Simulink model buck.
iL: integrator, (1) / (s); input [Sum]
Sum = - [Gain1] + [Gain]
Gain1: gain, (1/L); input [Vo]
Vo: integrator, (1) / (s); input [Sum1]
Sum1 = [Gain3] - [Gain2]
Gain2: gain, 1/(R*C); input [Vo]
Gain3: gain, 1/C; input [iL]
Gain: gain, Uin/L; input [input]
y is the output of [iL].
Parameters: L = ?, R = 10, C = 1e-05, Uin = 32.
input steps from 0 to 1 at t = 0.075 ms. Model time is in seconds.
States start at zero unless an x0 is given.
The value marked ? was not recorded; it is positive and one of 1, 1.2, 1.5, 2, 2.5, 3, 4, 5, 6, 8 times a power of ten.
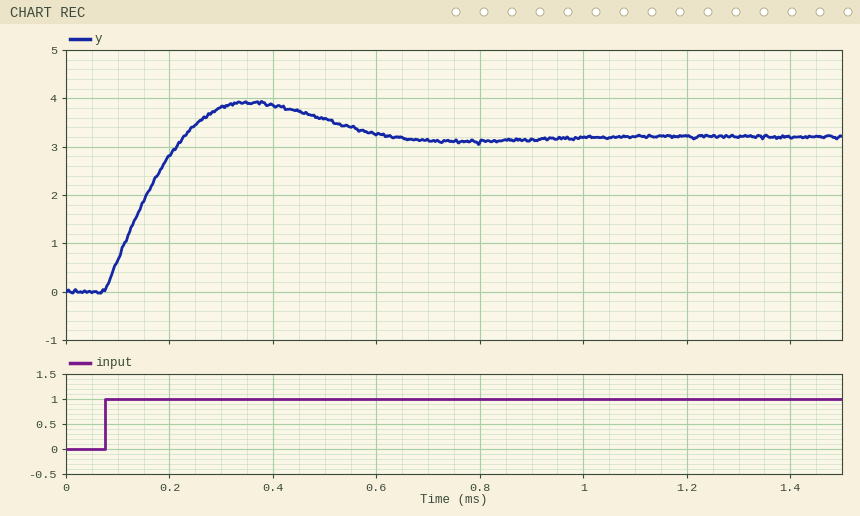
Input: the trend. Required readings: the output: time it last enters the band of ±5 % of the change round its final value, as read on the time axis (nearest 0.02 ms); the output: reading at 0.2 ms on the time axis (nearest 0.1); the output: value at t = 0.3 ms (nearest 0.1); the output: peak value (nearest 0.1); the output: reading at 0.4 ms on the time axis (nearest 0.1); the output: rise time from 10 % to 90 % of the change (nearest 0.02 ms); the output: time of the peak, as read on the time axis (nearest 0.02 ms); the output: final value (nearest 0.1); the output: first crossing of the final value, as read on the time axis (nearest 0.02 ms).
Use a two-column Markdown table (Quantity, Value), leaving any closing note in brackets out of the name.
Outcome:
| Quantity | Value |
|---|---|
| the output: time it last enters the band of ±5 % of the change round its final value, as read on the time axis | 0.56 ms |
| the output: reading at 0.2 ms on the time axis | 2.8 |
| the output: value at t = 0.3 ms | 3.8 |
| the output: peak value | 3.9 |
| the output: reading at 0.4 ms on the time axis | 3.9 |
| the output: rise time from 10 % to 90 % of the change | 0.12 ms |
| the output: time of the peak, as read on the time axis | 0.36 ms |
| the output: final value | 3.2 |
| the output: first crossing of the final value, as read on the time axis | 0.22 ms |
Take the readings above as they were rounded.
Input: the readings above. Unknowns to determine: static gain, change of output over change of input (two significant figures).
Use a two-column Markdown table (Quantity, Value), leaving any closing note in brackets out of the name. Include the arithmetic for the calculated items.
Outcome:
| Quantity | Value |
|---|---|
| static gain, change of output over change of input | (3.2 - 0) / (1 - 0) = 3.2 |
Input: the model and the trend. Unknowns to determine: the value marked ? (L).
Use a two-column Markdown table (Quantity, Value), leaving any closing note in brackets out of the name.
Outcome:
| Quantity | Value |
|---|---|
| the value marked ? | 0.0012 |
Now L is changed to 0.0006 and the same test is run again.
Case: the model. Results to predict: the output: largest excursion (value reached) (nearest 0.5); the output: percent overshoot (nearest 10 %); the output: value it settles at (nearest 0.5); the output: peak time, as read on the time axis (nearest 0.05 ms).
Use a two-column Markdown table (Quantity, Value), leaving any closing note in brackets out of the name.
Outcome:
| Quantity | Value |
|---|---|
| the output: largest excursion (value reached) | 5.0 |
| the output: percent overshoot | 60 % |
| the output: value it settles at | 3.0 |
| the output: peak time, as read on the time axis | 0.25 ms |
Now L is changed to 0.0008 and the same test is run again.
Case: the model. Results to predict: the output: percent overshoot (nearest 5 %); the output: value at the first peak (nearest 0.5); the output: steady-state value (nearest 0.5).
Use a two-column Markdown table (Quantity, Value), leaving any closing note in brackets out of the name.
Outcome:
| Quantity | Value |
|---|---|
| the output: percent overshoot | 40 % |
| the output: value at the first peak | 4.5 |
| the output: steady-state value | 3.0 |
